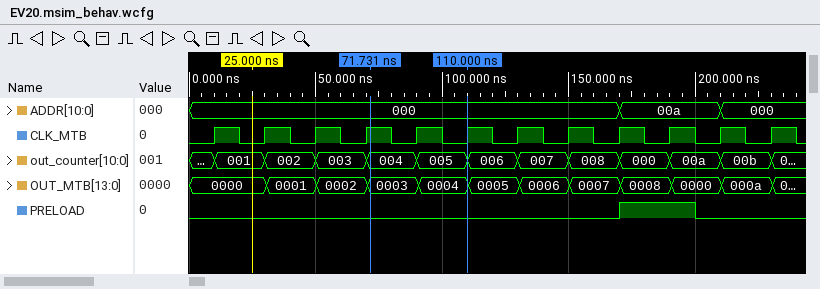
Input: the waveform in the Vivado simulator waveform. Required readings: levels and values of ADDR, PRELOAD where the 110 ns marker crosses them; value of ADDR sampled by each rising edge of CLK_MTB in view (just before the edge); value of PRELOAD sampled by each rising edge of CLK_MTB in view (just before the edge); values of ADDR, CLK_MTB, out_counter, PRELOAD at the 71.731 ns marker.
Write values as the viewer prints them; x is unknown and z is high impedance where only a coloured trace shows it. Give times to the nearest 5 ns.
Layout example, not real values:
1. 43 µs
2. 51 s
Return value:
1. ADDR=000, PRELOAD=0
2. 000, 000, 000, 000, 000, 000, 000, 000, 000, 00a, 00a, 000
3. 0 0 0 0 0 0 0 0 0 1 0 0
4. ADDR=000, CLK_MTB=1, out_counter=004, PRELOAD=0
